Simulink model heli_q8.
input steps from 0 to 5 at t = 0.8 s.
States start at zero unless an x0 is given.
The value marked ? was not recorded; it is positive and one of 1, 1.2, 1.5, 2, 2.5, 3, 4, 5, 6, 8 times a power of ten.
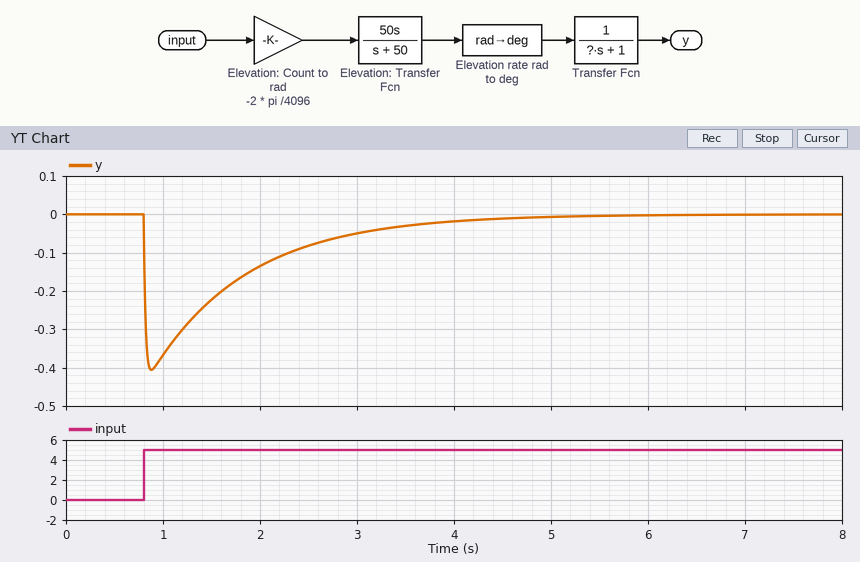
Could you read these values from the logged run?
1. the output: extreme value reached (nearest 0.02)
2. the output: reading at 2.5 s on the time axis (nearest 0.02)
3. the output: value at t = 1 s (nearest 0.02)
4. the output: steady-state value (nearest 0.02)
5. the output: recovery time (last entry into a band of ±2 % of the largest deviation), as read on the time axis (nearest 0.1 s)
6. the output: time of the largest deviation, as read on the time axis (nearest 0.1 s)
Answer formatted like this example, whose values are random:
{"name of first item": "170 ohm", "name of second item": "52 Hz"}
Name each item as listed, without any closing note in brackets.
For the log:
{"the output: extreme value reached": "-0.40", "the output: reading at 2.5 s on the time axis": "-0.08", "the output: value at t = 1 s": "-0.36", "the output: steady-state value": "0.00", "the output: recovery time (last entry into a band of ±2 % of the largest deviation), as read on the time axis": "4.8 s", "the output: time of the largest deviation, as read on the time axis": "0.9 s"}
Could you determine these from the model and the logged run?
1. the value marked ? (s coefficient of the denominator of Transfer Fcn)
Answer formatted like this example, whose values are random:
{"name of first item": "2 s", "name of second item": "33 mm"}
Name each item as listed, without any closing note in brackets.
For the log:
{"the value marked ?": "1"}
